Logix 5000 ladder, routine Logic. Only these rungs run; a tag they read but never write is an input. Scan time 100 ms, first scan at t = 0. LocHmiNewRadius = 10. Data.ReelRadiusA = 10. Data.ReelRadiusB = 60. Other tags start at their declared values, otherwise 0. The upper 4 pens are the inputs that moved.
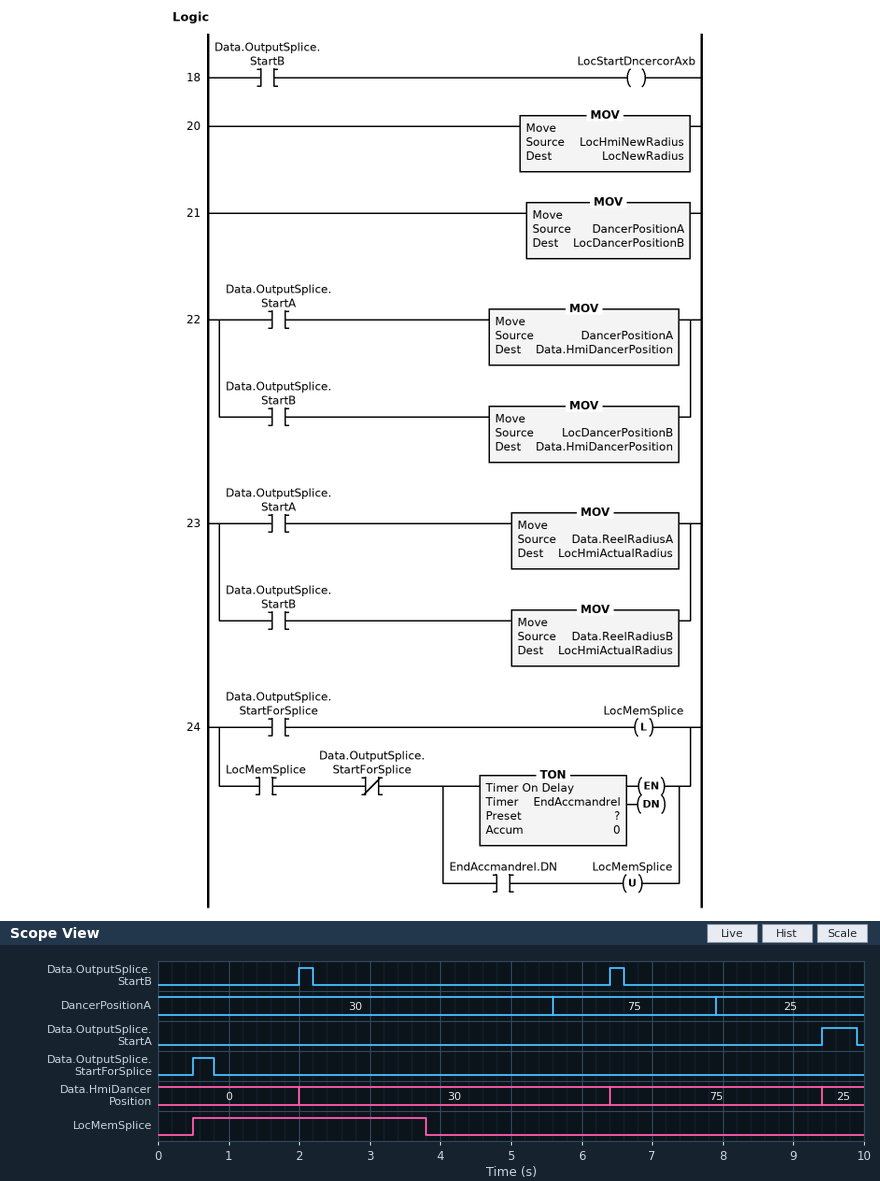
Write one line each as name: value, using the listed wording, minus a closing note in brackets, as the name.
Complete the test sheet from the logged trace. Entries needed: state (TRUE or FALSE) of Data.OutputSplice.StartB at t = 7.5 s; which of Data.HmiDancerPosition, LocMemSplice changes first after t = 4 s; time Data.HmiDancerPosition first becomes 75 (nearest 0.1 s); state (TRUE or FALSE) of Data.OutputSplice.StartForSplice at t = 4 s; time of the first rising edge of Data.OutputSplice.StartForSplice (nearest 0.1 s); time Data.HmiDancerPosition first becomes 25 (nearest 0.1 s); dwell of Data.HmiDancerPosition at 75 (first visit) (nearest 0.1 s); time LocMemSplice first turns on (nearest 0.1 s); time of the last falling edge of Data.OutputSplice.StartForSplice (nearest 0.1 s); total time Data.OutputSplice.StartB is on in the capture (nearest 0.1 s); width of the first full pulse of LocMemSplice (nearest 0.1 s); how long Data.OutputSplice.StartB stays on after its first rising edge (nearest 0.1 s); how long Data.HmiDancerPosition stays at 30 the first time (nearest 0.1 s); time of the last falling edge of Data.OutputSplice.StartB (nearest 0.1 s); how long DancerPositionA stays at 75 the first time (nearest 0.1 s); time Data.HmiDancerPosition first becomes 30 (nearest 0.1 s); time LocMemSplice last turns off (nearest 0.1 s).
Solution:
state (TRUE or FALSE) of Data.OutputSplice.StartB at t = 7.5 s: FALSE
which of Data.HmiDancerPosition, LocMemSplice changes first after t = 4 s: Data.HmiDancerPosition
time Data.HmiDancerPosition first becomes 75: 6.4 s
state (TRUE or FALSE) of Data.OutputSplice.StartForSplice at t = 4 s: FALSE
time of the first rising edge of Data.OutputSplice.StartForSplice: 0.5 s
time Data.HmiDancerPosition first becomes 25: 9.4 s
dwell of Data.HmiDancerPosition at 75 (first visit): 3.0 s
time LocMemSplice first turns on: 0.5 s
time of the last falling edge of Data.OutputSplice.StartForSplice: 0.8 s
total time Data.OutputSplice.StartB is on in the capture: 0.4 s
width of the first full pulse of LocMemSplice: 3.3 s
how long Data.OutputSplice.StartB stays on after its first rising edge: 0.2 s
how long Data.HmiDancerPosition stays at 30 the first time: 4.4 s
time of the last falling edge of Data.OutputSplice.StartB: 6.6 s
how long DancerPositionA stays at 75 the first time: 2.3 s
time Data.HmiDancerPosition first becomes 30: 2.0 s
time LocMemSplice last turns off: 3.8 s
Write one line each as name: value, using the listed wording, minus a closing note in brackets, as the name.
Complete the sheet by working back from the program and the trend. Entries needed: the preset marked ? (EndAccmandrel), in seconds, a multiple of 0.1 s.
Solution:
the preset marked ? (EndAccmandrel), in seconds, a multiple of 0.1 s: 3.0 s
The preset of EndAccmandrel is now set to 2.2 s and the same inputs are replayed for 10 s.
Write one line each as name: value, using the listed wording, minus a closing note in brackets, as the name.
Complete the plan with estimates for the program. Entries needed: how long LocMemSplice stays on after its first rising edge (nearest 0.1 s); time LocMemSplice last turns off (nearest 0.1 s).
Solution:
how long LocMemSplice stays on after its first rising edge: 2.5 s
time LocMemSplice last turns off: 3.0 s
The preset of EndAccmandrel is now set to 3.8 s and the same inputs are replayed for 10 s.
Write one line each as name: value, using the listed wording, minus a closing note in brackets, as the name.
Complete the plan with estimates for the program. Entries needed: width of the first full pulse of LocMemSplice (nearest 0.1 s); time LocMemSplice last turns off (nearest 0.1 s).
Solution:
width of the first full pulse of LocMemSplice: 4.1 s
time LocMemSplice last turns off: 4.6 s
